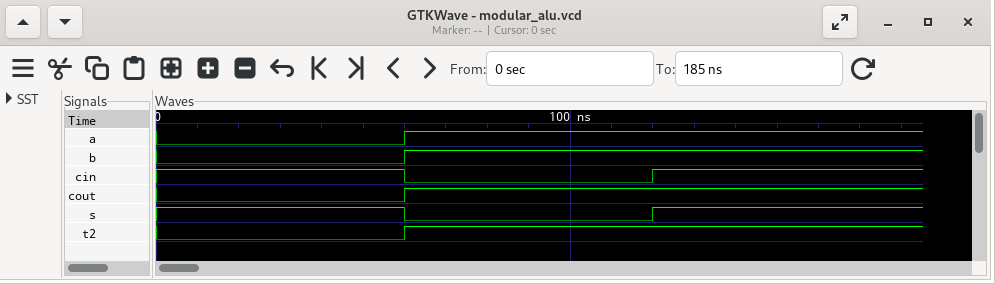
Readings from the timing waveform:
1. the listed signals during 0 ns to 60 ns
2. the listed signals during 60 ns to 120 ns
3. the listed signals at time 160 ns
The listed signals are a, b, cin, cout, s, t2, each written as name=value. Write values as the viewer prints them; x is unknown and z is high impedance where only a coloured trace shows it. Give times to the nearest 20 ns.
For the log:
a=0, b=0, cin=1, cout=0, s=1, t2=0
a=1, b=1, cin=0, cout=1, s=0, t2=1
a=1, b=1, cin=1, cout=1, s=1, t2=1
